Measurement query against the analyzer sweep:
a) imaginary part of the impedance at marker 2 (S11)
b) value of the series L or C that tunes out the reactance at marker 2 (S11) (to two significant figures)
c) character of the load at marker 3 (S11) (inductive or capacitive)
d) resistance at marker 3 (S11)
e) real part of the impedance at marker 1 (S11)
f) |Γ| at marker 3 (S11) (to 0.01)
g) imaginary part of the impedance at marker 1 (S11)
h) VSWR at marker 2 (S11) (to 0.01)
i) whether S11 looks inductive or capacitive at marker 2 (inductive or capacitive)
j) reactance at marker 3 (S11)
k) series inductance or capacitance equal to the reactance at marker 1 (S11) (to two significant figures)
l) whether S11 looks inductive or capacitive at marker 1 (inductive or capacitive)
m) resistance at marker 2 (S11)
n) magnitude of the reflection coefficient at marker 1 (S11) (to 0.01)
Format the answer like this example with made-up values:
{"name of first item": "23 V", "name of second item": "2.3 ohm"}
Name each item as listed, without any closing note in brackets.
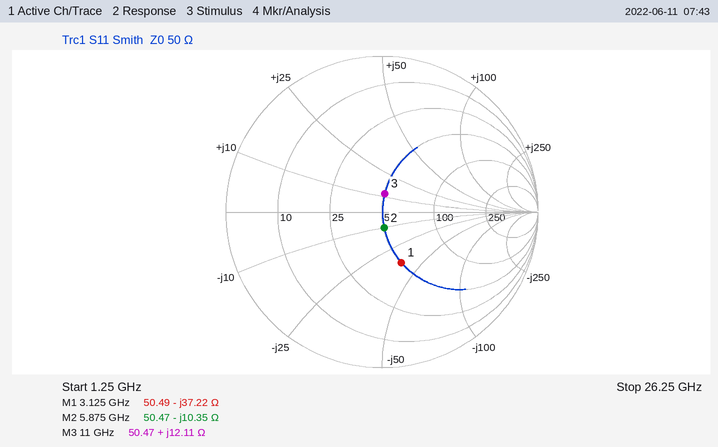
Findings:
{"imaginary part of the impedance at marker 2": "-10.35 Ω", "value of the series L or C that tunes out the reactance at marker 2 (S11)": "280 pH", "character of the load at marker 3 (S11)": "inductive", "resistance at marker 3": "50.47 Ω", "real part of the impedance at marker 1": "50.49 Ω", "|Γ| at marker 3 (S11)": "0.12", "imaginary part of the impedance at marker 1": "-37.22 Ω", "VSWR at marker 2 (S11)": "1.23", "whether S11 looks inductive or capacitive at marker 2": "capacitive", "reactance at marker 3": "+12.11 Ω", "series inductance or capacitance equal to the reactance at marker 1 (S11)": "1.4 pF", "whether S11 looks inductive or capacitive at marker 1": "capacitive", "resistance at marker 2": "50.47 Ω", "magnitude of the reflection coefficient at marker 1 (S11)": "0.35"}
